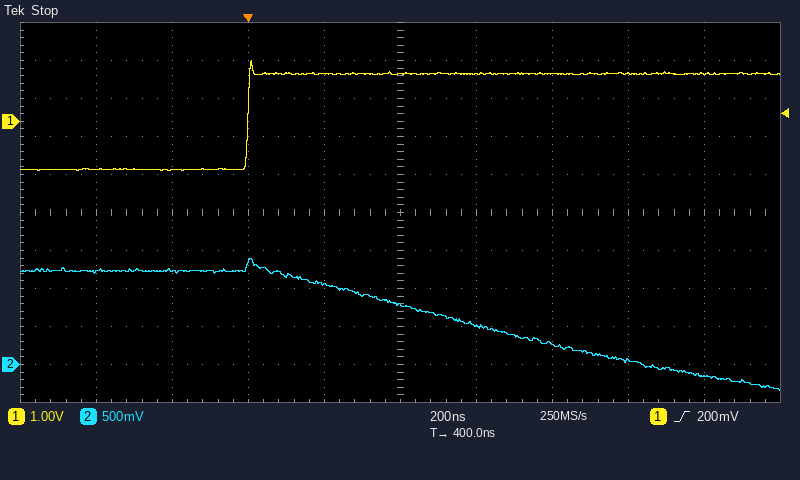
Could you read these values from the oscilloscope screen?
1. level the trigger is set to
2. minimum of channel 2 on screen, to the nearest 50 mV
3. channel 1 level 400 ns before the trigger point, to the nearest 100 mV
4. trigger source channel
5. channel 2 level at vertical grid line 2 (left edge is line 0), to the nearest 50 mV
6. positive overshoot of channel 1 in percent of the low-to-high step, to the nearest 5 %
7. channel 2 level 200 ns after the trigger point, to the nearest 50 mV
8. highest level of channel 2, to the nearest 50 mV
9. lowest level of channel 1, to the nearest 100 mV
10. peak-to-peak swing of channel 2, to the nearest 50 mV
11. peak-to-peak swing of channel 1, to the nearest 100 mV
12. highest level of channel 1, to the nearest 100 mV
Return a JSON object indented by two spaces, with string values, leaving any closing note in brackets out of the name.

{
  "level the trigger is set to": "200 mV",
  "minimum of channel 2 on screen, to the nearest 50 mV": "-350 mV",
  "channel 1 level 400 ns before the trigger point, to the nearest 100 mV": "-1.3 V",
  "trigger source channel": "channel 1",
  "channel 2 level at vertical grid line 2 (left edge is line 0), to the nearest 50 mV": "1.25 V",
  "positive overshoot of channel 1 in percent of the low-to-high step, to the nearest 5 %": "15 %",
  "channel 2 level 200 ns after the trigger point, to the nearest 50 mV": "1.05 V",
  "highest level of channel 2, to the nearest 50 mV": "1.40 V",
  "lowest level of channel 1, to the nearest 100 mV": "-1.3 V",
  "peak-to-peak swing of channel 2, to the nearest 50 mV": "1.75 V",
  "peak-to-peak swing of channel 1, to the nearest 100 mV": "2.9 V",
  "highest level of channel 1, to the nearest 100 mV": "1.6 V"
}
